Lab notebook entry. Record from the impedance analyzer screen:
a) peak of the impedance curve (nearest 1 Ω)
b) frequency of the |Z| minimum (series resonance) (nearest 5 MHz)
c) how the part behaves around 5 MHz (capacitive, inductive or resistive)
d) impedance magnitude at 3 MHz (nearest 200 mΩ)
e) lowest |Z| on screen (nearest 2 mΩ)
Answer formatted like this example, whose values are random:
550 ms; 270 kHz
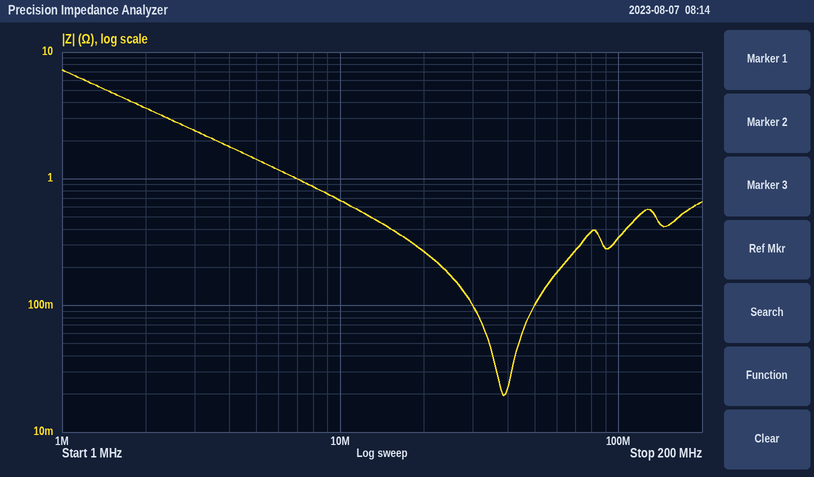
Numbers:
7 Ω; 40 MHz; capacitive; 2.4 Ω; 20 mΩ
